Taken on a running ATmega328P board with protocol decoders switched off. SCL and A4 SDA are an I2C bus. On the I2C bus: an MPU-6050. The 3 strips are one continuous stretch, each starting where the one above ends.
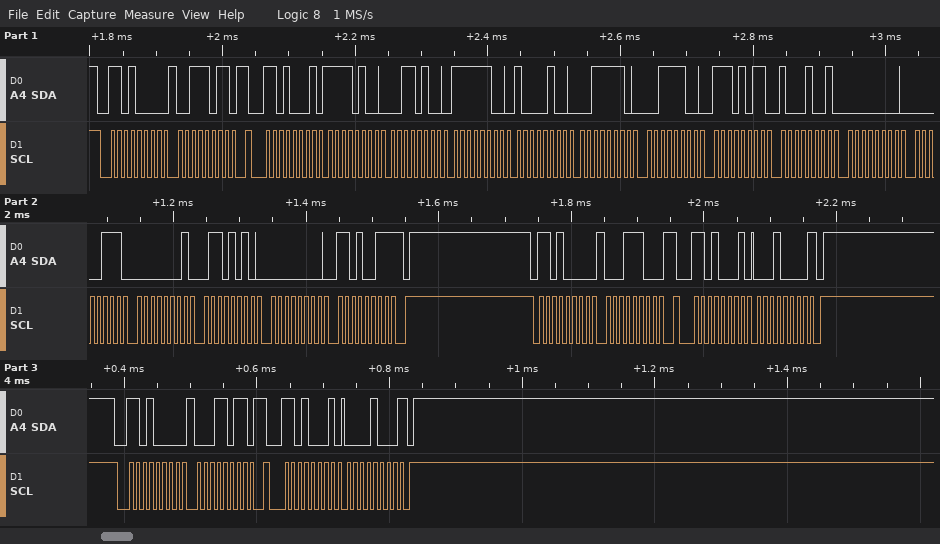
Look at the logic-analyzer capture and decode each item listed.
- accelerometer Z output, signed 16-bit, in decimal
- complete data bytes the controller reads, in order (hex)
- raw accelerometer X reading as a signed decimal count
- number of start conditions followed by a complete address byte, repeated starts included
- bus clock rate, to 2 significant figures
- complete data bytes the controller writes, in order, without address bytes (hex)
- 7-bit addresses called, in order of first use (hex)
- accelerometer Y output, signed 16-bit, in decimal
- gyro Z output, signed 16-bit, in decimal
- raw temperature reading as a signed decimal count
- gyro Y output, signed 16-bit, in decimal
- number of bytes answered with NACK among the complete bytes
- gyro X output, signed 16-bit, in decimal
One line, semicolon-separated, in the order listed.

15932; F4 34 FC 84 3E 3C EB 89 00 07 01 6A 00 D3 10 08; -3020; 6; 100 kHz; 3B 1C 1B; 0x68; -892; 211; -5239; 362; 3; 7
